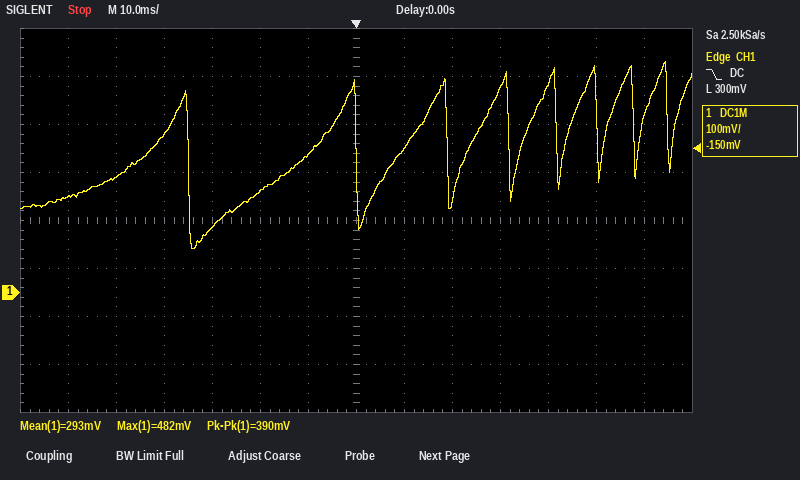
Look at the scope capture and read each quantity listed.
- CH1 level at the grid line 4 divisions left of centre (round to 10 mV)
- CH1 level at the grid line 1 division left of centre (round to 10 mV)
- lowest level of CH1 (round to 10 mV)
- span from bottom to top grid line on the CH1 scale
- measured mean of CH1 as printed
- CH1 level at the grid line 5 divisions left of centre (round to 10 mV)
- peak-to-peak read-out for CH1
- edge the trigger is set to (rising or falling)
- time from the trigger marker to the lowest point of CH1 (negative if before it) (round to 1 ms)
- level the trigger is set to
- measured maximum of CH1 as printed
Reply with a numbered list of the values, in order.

1. 330 mV
2. 290 mV
3. 90 mV
4. 800 mV
5. 293 mV
6. 240 mV
7. 390 mV
8. falling
9. -34 ms
10. 300 mV
11. 482 mV
